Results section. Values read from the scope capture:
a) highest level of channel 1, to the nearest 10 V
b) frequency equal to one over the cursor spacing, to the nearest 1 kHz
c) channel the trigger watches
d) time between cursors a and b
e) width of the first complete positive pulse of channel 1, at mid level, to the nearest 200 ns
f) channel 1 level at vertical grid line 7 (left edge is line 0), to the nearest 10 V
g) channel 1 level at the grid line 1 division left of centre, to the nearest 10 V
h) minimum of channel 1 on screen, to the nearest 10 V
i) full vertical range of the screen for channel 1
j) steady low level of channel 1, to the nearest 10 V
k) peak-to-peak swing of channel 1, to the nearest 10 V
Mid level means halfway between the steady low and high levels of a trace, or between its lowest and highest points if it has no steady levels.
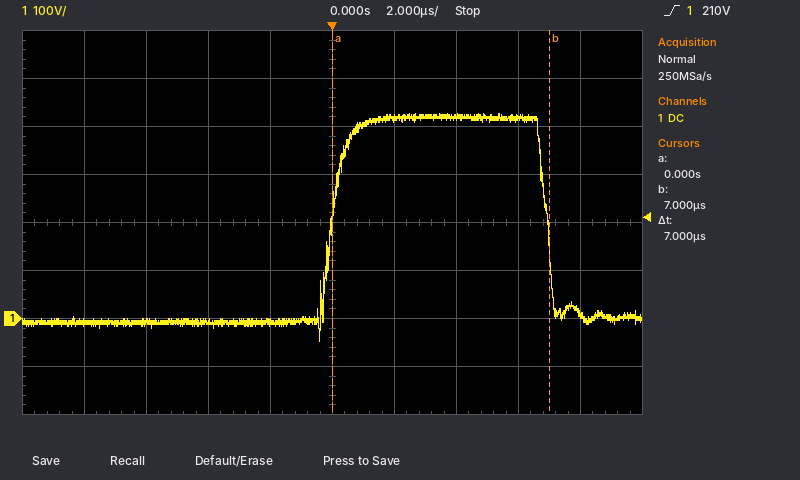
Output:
430 V
143 kHz
channel 1
7 µs
7.0 µs
420 V
-10 V
-50 V
800 V
-10 V
480 V
